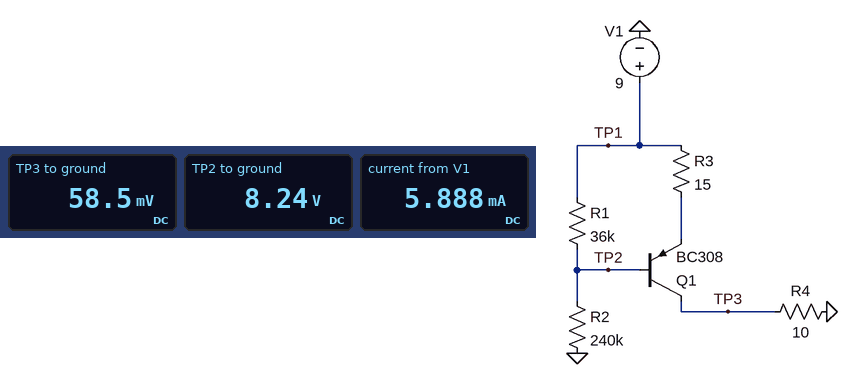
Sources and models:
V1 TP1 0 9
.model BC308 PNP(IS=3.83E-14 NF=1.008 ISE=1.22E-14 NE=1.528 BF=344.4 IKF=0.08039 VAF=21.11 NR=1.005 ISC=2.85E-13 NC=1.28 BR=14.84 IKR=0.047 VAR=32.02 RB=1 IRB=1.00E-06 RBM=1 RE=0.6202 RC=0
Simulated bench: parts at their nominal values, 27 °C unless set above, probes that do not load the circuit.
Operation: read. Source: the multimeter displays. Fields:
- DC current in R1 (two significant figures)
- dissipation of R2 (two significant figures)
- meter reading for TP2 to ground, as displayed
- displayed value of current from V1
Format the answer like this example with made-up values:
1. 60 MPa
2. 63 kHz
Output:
1. 21 µA
2. 280 µW
3. 8.24 V
4. 5.888 mA
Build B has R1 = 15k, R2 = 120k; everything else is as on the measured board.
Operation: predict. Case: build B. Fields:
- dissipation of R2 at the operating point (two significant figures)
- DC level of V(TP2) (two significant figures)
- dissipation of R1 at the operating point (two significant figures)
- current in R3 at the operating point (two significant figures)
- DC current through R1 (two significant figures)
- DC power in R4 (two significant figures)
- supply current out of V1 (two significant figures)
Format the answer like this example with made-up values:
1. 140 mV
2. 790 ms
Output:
1. 560 µW
2. 8.2 V
3. 41 µW
4. 7.1 mA
5. 52 µA
6. 510 µW
7. 7.2 mA
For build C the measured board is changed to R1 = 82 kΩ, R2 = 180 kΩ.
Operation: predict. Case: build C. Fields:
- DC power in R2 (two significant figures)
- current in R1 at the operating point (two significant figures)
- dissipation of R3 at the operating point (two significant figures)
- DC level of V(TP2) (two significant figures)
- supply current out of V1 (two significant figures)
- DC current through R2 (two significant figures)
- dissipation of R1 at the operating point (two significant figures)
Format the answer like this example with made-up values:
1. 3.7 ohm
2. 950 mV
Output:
1. 360 µW
2. 11 µA
3. 2.9 mW
4. 8.1 V
5. 14 mA
6. 45 µA
7. 10 µW
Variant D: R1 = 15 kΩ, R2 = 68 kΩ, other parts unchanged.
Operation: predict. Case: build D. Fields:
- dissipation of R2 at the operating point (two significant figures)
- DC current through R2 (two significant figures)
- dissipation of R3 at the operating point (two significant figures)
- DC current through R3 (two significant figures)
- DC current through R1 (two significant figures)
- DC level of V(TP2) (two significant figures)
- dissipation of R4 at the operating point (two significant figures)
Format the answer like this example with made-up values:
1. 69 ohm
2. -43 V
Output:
1. 940 µW
2. 120 µA
3. 5.8 mW
4. 20 mA
5. 67 µA
6. 8.0 V
7. 3.8 mW
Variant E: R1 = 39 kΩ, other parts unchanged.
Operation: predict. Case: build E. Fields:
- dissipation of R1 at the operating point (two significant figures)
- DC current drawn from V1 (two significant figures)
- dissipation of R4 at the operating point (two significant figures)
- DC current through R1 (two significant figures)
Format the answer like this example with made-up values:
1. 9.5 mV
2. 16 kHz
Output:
1. 15 µW
2. 6.4 mA
3. 410 µW
4. 20 µA
